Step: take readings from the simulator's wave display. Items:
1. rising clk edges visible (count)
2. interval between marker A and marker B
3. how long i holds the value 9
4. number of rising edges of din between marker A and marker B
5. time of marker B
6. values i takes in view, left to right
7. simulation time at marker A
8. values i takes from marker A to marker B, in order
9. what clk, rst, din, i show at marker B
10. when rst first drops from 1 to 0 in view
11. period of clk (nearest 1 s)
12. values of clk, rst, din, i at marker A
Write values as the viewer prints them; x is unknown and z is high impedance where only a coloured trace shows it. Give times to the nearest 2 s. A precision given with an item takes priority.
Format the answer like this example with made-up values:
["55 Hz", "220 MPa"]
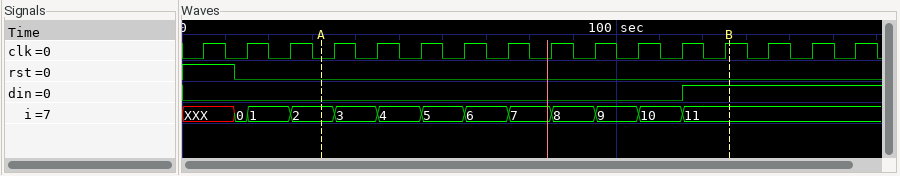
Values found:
["16", "94 s", "10 s", "1", "126 s", "XXX, 0, 1, 2, 3, 4, 5, 6, 7, 8, 9, 10, 11", "32 s", "2, 3, 4, 5, 6, 7, 8, 9, 10, 11", "clk=1, rst=0, din=1, i=11", "12 s", "10 s", "clk=0, rst=0, din=0, i=2"]
